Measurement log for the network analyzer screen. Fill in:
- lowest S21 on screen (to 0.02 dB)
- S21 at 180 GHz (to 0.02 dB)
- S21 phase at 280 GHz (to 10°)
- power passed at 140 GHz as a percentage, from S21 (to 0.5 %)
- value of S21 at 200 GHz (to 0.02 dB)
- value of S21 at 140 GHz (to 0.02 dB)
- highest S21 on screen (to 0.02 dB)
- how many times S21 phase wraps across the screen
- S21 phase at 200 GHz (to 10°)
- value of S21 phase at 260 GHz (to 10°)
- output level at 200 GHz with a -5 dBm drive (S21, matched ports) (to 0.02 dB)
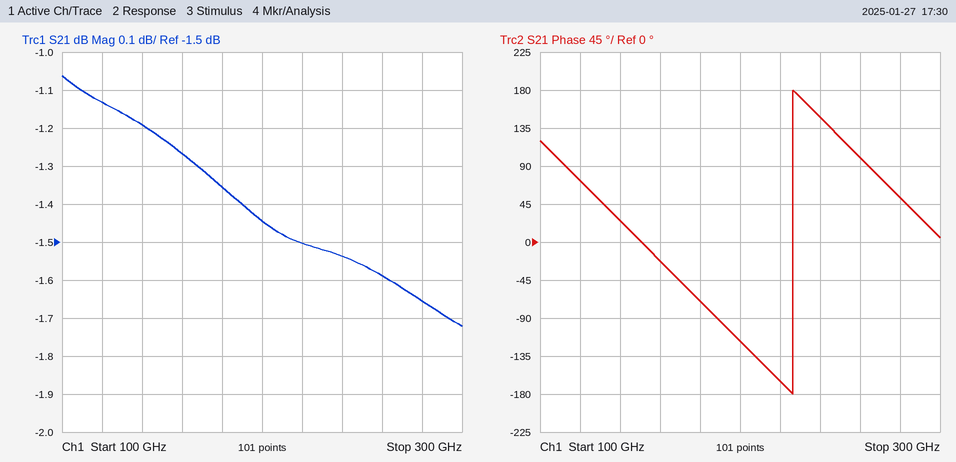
-1.72 dB
-1.36 dB
50°
76.0 %
-1.44 dB
-1.20 dB
-1.06 dB
1
-120°
100°
-6.44 dBm
